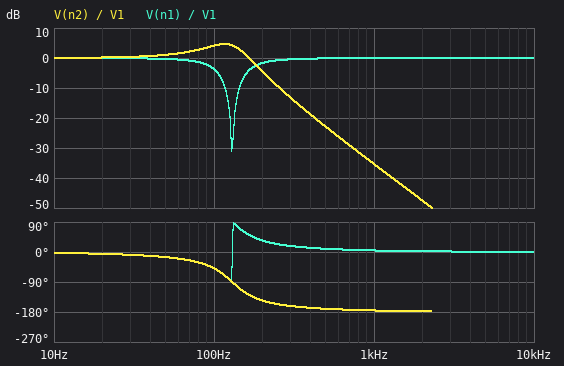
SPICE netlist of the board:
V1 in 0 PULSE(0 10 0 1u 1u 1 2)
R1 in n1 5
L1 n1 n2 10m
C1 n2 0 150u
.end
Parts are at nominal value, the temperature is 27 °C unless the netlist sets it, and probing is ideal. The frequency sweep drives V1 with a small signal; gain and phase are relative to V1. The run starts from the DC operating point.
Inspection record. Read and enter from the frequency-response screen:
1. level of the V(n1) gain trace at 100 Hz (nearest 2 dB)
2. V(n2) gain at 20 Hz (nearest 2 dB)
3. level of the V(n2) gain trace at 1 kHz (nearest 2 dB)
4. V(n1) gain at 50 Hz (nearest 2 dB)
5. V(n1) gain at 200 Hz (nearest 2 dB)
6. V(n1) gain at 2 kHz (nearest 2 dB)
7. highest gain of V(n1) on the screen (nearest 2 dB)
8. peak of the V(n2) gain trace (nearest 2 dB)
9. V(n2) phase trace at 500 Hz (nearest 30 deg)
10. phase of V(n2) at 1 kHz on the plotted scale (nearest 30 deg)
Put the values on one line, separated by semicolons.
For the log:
-4 dB; 0 dB; -36 dB; 0 dB; -2 dB; 0 dB; 0 dB; 4 dB; -180 deg; -180 deg
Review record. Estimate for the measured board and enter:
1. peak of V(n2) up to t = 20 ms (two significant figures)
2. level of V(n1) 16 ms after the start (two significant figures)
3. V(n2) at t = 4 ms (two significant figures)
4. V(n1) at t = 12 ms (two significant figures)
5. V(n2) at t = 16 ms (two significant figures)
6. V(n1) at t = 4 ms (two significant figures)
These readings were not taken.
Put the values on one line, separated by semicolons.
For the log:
14 V; 10 V; 14 V; 10 V; 9.8 V; 9.9 V
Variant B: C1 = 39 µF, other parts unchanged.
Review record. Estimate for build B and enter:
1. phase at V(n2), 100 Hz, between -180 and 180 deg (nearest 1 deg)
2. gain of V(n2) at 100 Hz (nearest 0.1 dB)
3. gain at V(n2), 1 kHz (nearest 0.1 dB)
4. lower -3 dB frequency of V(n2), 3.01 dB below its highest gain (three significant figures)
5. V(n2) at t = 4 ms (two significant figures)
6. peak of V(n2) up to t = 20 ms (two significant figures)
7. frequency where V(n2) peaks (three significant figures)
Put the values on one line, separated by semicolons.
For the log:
-8 deg; 1.4 dB; -23.2 dB; 204 Hz; 6.3 V; 16 V; 249 Hz
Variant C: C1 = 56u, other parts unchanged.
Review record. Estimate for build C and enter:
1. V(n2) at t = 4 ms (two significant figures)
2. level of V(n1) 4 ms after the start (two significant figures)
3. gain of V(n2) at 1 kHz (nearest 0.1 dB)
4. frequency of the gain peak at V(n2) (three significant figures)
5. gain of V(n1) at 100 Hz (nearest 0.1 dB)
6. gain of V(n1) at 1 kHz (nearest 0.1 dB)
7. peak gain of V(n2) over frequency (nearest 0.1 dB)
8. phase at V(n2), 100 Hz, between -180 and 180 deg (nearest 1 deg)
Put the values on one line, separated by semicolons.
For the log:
8.7 V; 11 V; -26.5 dB; 205 Hz; -0.2 dB; 0 dB; 8.7 dB; -13 deg
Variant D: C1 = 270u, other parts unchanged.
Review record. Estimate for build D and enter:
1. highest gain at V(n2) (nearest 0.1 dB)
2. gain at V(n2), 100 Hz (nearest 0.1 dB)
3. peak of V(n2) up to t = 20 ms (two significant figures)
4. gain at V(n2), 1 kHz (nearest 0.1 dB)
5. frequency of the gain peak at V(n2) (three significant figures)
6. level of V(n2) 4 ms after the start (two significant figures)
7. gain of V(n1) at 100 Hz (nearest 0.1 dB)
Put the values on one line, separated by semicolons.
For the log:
2.5 dB; 1.4 dB; 12 V; -40.5 dB; 78.8 Hz; 11 V; -22.2 dB
